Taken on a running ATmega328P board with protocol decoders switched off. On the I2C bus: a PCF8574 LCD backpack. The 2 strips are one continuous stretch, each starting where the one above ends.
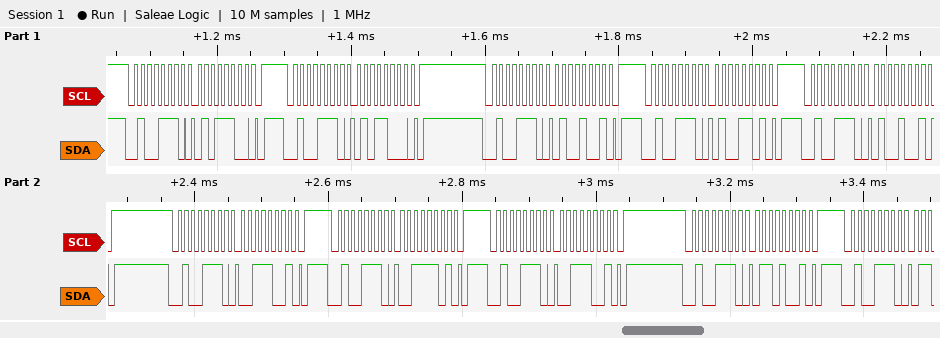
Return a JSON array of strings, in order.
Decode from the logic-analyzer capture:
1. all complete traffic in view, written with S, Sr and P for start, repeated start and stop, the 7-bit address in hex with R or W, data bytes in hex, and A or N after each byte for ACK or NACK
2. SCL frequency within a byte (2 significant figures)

["S 27W A 5C A P S 27W A 58 A P S 27W A 49 A P S 27W A 4D A P S 27W A 49 A P S 27W A 39 A P S 27W A 3D A P S 27W A 39 A P S 27W A 69 A P S 27W A", "100 kHz"]
